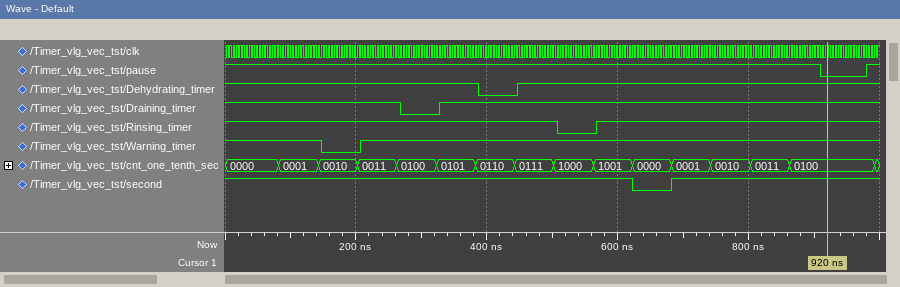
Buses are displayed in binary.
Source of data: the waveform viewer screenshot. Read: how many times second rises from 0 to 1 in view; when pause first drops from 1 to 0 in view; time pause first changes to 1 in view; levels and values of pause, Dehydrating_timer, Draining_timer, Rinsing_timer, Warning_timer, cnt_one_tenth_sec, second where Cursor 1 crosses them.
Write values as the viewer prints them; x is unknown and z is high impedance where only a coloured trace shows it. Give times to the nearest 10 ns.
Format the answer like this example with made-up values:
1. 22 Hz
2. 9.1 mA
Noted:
1. 1
2. 910 ns
3. 980 ns
4. pause=0, Dehydrating_timer=1, Draining_timer=1, Rinsing_timer=1, Warning_timer=1, cnt_one_tenth_sec=0100, second=1
